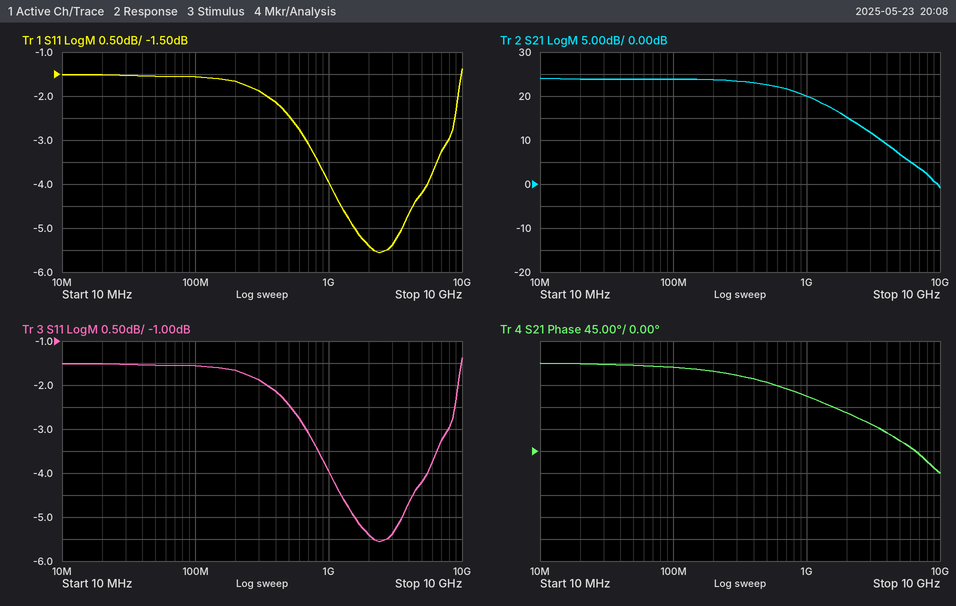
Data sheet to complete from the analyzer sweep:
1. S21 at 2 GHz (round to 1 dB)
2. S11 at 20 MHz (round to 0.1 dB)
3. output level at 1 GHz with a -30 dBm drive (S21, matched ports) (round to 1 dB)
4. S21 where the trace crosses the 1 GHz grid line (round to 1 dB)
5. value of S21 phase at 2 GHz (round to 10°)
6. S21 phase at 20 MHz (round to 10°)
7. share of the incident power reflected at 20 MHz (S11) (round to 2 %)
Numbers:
15 dB
-1.5 dB
-10 dBm
20 dB
80°
180°
70 %
